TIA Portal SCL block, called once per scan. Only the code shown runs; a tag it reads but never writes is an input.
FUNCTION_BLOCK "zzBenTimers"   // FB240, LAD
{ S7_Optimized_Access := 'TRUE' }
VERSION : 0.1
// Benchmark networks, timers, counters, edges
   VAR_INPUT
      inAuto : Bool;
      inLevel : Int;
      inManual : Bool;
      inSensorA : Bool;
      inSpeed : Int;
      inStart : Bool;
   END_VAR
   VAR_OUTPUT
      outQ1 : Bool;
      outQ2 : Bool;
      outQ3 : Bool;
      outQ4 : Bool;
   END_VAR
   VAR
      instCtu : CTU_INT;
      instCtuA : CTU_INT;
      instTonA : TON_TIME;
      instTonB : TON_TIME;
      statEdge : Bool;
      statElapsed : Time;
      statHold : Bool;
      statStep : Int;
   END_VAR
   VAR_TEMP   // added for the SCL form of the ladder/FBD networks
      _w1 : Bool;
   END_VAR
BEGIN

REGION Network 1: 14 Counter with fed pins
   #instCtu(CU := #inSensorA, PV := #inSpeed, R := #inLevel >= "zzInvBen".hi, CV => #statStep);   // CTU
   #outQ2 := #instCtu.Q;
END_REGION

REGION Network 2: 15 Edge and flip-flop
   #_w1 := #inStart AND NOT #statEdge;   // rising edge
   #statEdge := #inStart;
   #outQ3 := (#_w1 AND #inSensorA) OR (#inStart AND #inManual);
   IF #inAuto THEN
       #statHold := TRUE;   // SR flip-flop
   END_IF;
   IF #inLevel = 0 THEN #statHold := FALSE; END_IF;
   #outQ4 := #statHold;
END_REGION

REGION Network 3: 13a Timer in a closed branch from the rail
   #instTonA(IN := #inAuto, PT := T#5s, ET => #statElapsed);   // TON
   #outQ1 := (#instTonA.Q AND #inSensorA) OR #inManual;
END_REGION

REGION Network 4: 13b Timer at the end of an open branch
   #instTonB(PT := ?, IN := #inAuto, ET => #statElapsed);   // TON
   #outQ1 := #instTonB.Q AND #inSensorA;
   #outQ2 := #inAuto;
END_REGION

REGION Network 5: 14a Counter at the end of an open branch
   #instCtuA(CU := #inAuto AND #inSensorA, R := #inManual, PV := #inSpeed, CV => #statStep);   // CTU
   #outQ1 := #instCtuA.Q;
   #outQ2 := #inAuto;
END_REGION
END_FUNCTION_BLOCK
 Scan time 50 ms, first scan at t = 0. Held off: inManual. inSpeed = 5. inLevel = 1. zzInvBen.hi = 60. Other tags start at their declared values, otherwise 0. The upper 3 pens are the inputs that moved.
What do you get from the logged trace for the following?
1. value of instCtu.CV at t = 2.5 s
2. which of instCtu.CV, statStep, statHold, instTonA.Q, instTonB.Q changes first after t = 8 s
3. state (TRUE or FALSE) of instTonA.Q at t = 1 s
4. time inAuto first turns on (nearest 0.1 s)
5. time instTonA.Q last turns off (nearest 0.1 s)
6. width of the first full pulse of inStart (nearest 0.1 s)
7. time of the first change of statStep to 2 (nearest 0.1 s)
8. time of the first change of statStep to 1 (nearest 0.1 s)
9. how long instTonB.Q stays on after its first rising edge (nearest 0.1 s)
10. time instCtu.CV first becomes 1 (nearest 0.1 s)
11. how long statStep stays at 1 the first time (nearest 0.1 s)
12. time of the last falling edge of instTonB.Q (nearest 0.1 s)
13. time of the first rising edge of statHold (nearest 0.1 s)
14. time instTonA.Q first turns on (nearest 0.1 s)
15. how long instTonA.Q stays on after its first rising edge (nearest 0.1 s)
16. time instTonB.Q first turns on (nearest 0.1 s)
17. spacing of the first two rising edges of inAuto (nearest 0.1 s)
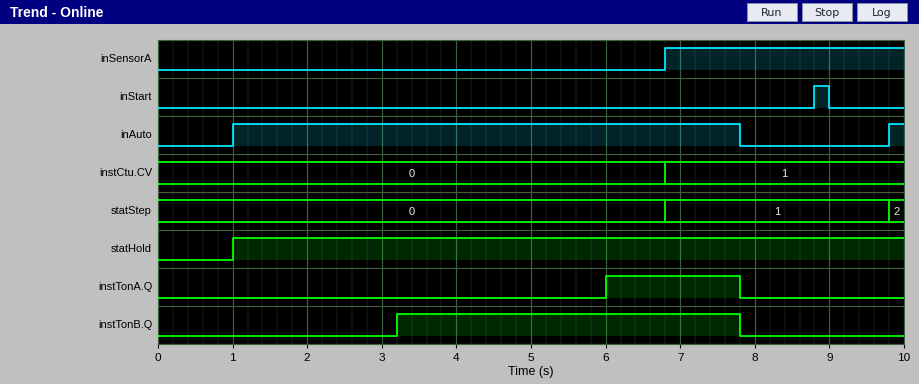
0
statStep
FALSE
1.0 s
7.8 s
0.2 s
9.8 s
6.8 s
4.6 s
6.8 s
3.0 s
7.8 s
1.0 s
6.0 s
1.8 s
3.2 s
8.8 s
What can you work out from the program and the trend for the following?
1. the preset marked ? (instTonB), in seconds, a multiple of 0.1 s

2.2 s
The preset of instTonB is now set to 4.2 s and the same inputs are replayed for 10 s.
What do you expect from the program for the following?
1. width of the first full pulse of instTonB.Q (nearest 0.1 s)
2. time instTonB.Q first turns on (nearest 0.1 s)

2.6 s
5.2 s
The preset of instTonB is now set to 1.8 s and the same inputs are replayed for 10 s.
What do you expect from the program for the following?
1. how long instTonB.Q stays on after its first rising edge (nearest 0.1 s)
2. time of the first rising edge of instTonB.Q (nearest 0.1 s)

5.0 s
2.8 s
